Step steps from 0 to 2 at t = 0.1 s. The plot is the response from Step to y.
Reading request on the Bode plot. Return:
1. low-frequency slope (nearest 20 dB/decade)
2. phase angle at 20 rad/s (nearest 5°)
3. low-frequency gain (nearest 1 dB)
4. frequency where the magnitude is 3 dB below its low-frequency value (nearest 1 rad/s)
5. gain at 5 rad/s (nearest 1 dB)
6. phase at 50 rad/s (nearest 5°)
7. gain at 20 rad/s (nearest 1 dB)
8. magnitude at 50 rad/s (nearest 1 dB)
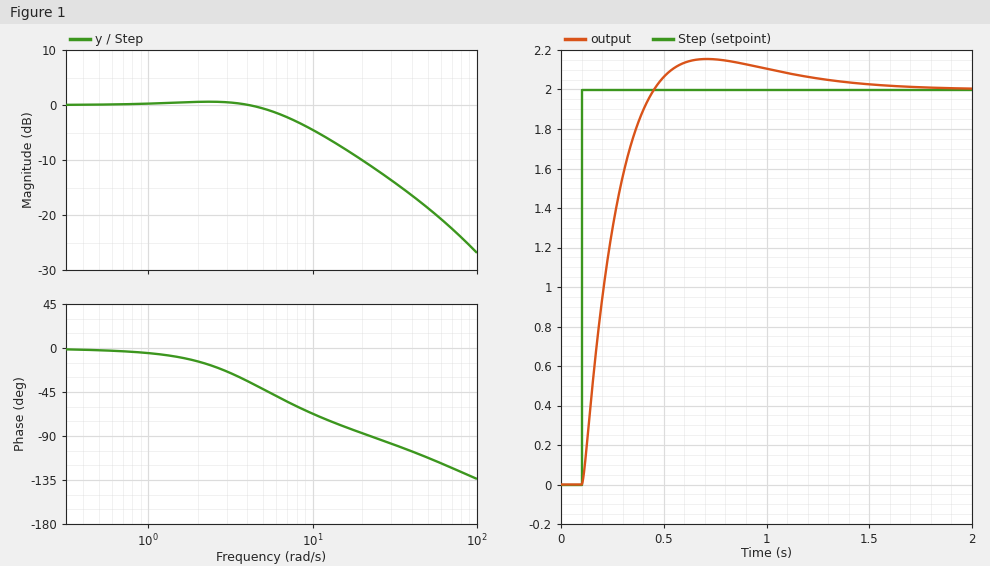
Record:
0 dB/decade
-85°
0 dB
8 rad/s
-1 dB
-110°
-10 dB
-19 dB
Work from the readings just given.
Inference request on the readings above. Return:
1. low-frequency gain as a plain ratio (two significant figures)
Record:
1.0
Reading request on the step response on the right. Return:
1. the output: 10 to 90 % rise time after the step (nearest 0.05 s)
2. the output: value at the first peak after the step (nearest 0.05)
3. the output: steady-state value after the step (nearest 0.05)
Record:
0.25 s
2.15
2.00
